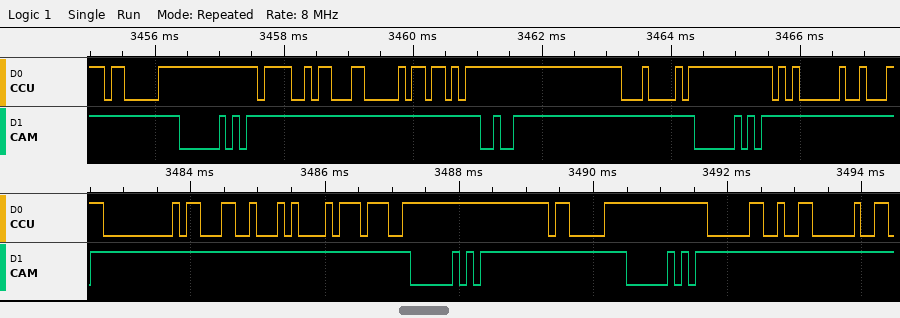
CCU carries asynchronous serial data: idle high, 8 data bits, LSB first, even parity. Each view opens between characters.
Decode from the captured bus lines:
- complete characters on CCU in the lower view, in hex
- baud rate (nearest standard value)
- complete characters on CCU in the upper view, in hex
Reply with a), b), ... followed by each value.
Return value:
a) 00, 63, 14, 77, 83, 60, 06
b) 9600 baud
c) 83, 4F, 0C, 5B, 84, 05
